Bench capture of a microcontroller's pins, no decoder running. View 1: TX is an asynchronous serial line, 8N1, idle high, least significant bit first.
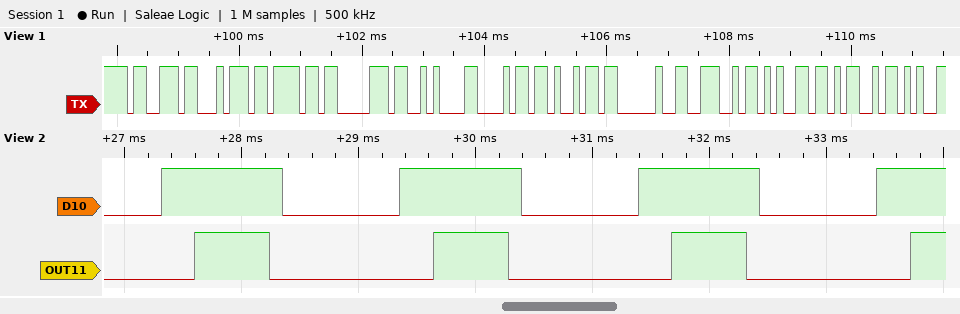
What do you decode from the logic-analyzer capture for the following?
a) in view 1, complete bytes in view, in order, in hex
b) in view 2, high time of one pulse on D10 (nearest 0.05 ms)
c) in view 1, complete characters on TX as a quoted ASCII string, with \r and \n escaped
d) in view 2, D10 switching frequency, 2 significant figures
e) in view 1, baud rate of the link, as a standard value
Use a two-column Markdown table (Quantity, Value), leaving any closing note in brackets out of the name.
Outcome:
| Quantity | Value |
|---|---|
| in view 1, complete bytes in view, in order, in hex | 73 74 6F 70 0A 68 69 20 4E 65 4D |
| in view 2, high time of one pulse on D10 | 1.05 ms |
| in view 1, complete characters on TX as a quoted ASCII string, with \r and \n escaped | "stop\nhi NeM" |
| in view 2, D10 switching frequency, 2 significant figures | 490 Hz |
| in view 1, baud rate of the link, as a standard value | 9600 baud |
